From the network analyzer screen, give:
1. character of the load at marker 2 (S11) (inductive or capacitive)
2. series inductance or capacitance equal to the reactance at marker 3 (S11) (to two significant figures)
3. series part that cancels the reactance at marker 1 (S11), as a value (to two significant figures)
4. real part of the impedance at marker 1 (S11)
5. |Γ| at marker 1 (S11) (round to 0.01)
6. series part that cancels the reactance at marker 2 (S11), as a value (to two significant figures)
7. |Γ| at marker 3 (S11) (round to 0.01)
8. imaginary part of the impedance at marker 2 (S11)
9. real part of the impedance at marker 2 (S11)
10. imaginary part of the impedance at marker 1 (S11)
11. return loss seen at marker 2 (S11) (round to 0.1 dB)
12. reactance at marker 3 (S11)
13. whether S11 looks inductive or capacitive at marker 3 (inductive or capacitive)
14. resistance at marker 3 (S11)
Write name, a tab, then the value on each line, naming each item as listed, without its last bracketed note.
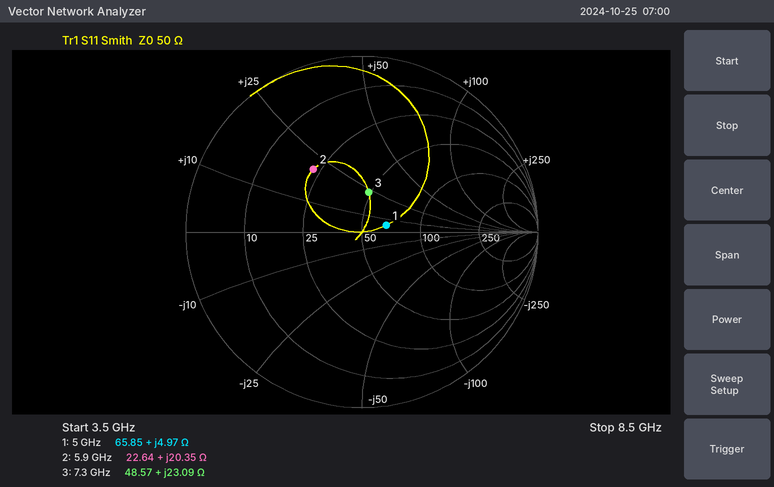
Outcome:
character of the load at marker 2 (S11)	inductive
series inductance or capacitance equal to the reactance at marker 3 (S11)	500 pH
series part that cancels the reactance at marker 1 (S11), as a value	6.4 pF
real part of the impedance at marker 1	65.85 Ω
|Γ| at marker 1 (S11)	0.14
series part that cancels the reactance at marker 2 (S11), as a value	1.3 pF
|Γ| at marker 3 (S11)	0.23
imaginary part of the impedance at marker 2	+20.35 Ω
real part of the impedance at marker 2	22.64 Ω
imaginary part of the impedance at marker 1	+4.97 Ω
return loss seen at marker 2 (S11)	6.9 dB
reactance at marker 3	+23.09 Ω
whether S11 looks inductive or capacitive at marker 3	inductive
resistance at marker 3	48.57 Ω
